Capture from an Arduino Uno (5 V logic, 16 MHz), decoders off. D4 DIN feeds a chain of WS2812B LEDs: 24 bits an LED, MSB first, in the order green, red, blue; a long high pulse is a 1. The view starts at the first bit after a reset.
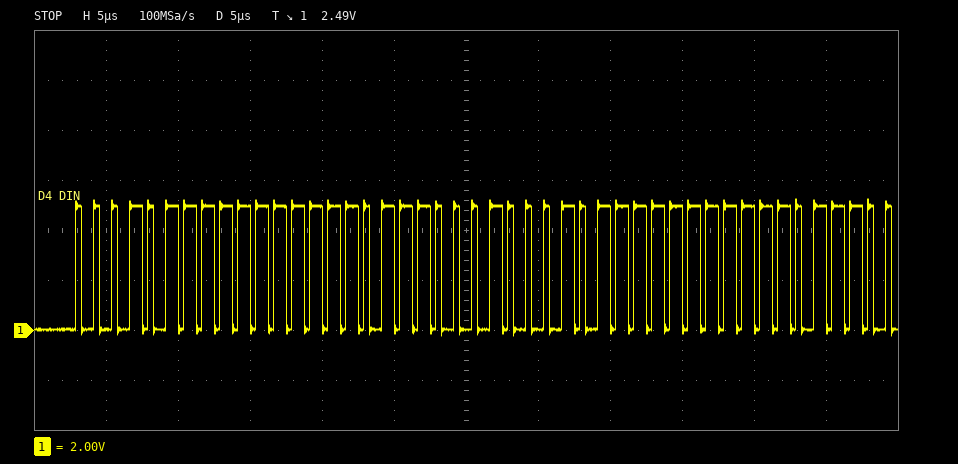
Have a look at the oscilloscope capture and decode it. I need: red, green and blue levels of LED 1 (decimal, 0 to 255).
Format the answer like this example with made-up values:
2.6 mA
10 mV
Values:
255, 23, 113
